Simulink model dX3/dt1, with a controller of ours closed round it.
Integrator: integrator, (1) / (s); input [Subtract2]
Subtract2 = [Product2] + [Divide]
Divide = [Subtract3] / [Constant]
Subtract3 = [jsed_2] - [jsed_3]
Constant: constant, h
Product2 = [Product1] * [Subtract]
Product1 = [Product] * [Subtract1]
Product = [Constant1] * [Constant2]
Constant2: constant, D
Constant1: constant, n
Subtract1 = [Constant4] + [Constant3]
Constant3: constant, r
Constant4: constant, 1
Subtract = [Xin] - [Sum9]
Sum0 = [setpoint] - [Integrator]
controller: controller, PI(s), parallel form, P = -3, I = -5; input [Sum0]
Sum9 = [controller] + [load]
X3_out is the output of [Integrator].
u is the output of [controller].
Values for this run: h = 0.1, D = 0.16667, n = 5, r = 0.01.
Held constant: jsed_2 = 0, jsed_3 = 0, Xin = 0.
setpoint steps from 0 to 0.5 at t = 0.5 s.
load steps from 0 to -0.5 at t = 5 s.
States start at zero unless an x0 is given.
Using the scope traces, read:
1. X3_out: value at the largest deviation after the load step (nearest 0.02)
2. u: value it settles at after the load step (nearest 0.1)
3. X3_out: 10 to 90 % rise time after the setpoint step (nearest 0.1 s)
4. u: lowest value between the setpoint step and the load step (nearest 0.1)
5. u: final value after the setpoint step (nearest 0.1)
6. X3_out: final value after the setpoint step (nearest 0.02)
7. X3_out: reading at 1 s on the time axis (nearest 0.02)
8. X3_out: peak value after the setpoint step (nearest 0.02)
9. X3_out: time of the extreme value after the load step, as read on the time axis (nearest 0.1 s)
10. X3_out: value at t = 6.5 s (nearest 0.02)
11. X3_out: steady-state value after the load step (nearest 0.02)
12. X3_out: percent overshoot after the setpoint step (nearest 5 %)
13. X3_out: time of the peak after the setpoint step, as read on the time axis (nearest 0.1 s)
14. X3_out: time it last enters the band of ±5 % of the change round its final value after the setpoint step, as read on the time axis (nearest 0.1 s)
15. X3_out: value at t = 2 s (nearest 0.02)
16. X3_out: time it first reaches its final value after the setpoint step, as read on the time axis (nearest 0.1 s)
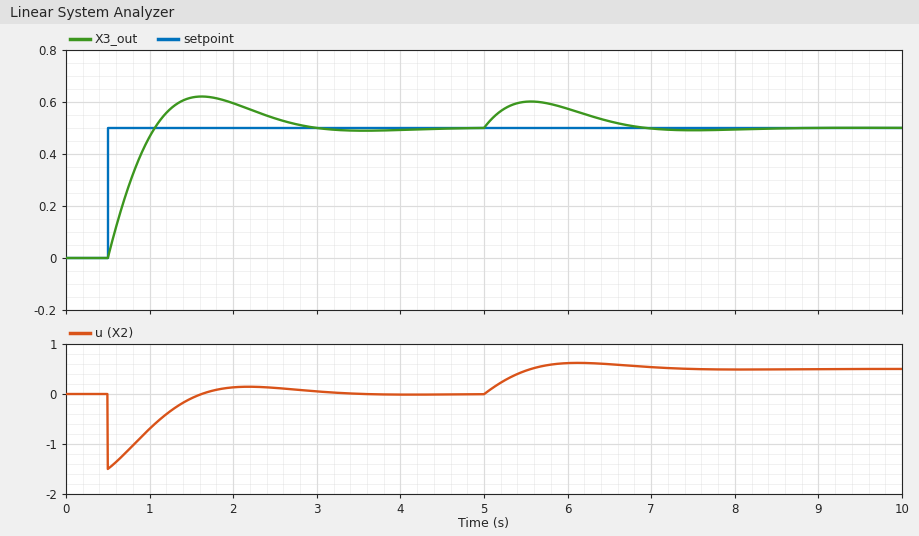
0.60
0.5
0.4 s
-1.5
0.0
0.50
0.46
0.62
5.6 s
0.52
0.50
25 %
1.6 s
2.6 s
0.60
1.1 s
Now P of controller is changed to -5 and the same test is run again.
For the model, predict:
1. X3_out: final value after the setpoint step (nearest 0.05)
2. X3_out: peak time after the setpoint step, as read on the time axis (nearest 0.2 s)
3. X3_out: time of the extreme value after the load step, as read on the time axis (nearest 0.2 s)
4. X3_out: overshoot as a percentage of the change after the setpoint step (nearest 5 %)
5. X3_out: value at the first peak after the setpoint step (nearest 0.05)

0.50
1.4 s
5.4 s
15 %
0.55
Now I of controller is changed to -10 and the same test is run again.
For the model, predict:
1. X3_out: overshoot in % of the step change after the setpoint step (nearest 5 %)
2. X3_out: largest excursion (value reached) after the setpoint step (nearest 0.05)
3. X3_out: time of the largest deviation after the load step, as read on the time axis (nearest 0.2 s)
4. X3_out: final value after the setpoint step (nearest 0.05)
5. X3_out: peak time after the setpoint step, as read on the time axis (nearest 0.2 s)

35 %
0.65
5.4 s
0.50
1.4 s
